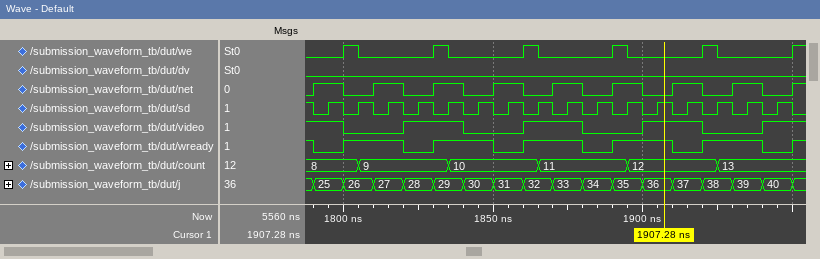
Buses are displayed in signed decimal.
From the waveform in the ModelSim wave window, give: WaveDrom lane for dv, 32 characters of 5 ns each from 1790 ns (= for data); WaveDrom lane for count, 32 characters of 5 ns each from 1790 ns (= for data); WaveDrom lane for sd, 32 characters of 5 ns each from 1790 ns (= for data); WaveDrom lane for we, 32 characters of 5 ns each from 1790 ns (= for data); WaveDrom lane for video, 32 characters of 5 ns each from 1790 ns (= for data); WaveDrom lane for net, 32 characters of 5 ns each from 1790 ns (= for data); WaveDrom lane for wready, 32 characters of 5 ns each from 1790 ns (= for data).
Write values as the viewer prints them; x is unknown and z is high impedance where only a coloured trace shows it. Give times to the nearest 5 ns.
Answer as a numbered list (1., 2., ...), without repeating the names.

1. {name: 'dv', wave: '0...............................'}
2. {name: 'count', wave: '=..=.....=.....=.....=.....=....', data: '8 9 10 11 12 13'}
3. {name: 'sd', wave: '01010101010101010101010101010101'}
4. {name: 'we', wave: '0.10....10....10....10....10....'}
5. {name: 'video', wave: '1.0...1...0...1...0...1...0...1.'}
6. {name: 'net', wave: '1.0.1.0.1.0.1.0.1.0.1.0.1.0.1.0.'}
7. {name: 'wready', wave: '0.1...0.1...0.1...0.1...0.1...0.'}
